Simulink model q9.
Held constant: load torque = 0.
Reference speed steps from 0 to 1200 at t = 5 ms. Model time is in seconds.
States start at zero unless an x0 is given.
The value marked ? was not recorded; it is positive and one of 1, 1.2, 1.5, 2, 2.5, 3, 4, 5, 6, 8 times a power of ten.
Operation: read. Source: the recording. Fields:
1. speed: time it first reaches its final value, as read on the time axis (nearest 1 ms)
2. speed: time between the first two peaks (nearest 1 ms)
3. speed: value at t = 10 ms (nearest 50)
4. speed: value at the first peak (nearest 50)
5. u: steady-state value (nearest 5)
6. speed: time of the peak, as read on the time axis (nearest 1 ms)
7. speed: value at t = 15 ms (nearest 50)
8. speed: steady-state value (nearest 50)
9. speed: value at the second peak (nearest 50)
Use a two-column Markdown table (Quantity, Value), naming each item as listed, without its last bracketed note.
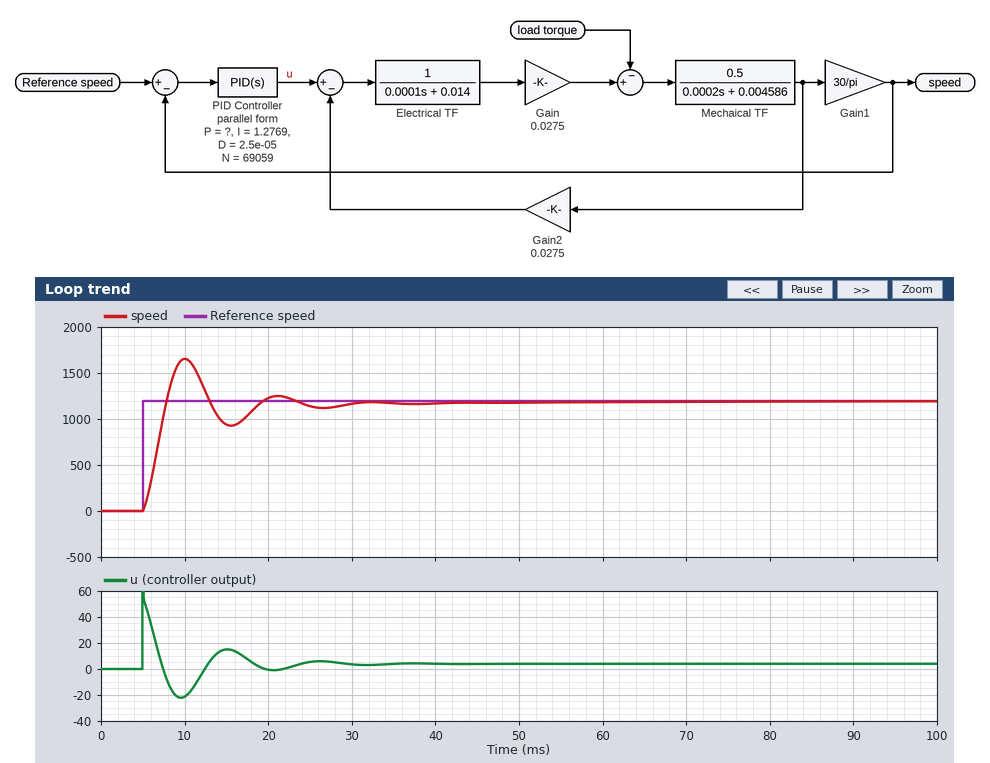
| Quantity | Value |
|---|---|
| speed: time it first reaches its final value, as read on the time axis | 8 ms |
| speed: time between the first two peaks | 11 ms |
| speed: value at t = 10 ms | 1650 |
| speed: value at the first peak | 1650 |
| u: steady-state value | 5 |
| speed: time of the peak, as read on the time axis | 10 ms |
| speed: value at t = 15 ms | 950 |
| speed: steady-state value | 1200 |
| speed: value at the second peak | 1250 |
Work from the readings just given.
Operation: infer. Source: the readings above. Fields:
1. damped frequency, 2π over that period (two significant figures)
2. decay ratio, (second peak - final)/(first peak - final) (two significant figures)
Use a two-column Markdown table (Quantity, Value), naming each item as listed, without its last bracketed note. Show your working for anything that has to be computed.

| Quantity | Value |
|---|---|
| damped frequency, 2π over that period | 2π / 11 = 0.57 rad/ms |
| decay ratio, (second peak - final)/(first peak - final) | (1250 - 1200) / (1650 - 1200) = 0.11 |
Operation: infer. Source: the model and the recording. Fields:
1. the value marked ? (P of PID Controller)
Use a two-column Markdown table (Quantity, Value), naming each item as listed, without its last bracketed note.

| Quantity | Value |
|---|---|
| the value marked ? | 0.05 |
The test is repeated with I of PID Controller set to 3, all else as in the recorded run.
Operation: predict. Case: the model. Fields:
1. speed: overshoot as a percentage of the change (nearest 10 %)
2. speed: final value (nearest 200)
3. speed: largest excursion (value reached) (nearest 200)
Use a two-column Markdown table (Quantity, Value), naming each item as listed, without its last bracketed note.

| Quantity | Value |
|---|---|
| speed: overshoot as a percentage of the change | 40 % |
| speed: final value | 1200 |
| speed: largest excursion (value reached) | 1800 |
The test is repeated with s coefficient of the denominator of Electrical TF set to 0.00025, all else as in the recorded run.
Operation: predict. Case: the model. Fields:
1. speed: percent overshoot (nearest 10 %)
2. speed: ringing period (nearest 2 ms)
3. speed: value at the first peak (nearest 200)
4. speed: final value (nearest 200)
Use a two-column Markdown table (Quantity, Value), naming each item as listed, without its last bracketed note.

| Quantity | Value |
|---|---|
| speed: percent overshoot | 50 % |
| speed: ringing period | 18 ms |
| speed: value at the first peak | 1800 |
| speed: final value | 1200 |
